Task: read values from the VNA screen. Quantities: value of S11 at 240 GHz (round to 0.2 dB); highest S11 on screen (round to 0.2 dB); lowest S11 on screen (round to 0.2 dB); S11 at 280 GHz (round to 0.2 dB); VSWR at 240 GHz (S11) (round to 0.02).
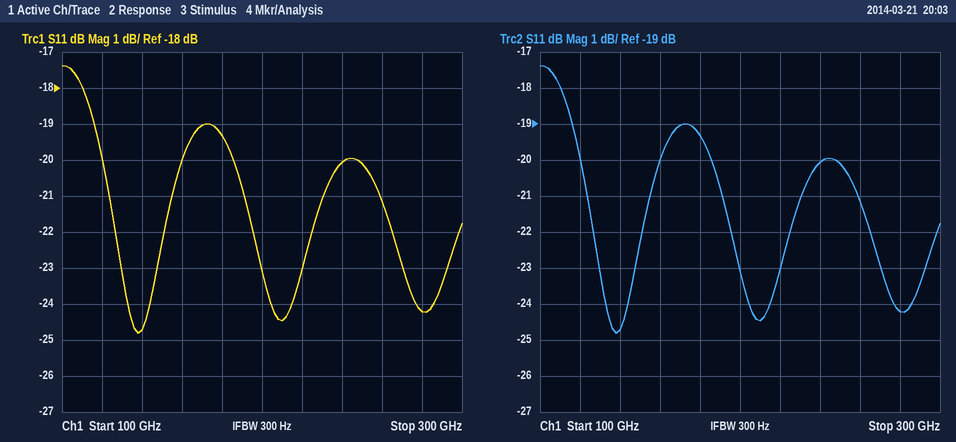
-20.0 dB
-17.4 dB
-24.8 dB
-24.2 dB
1.22
